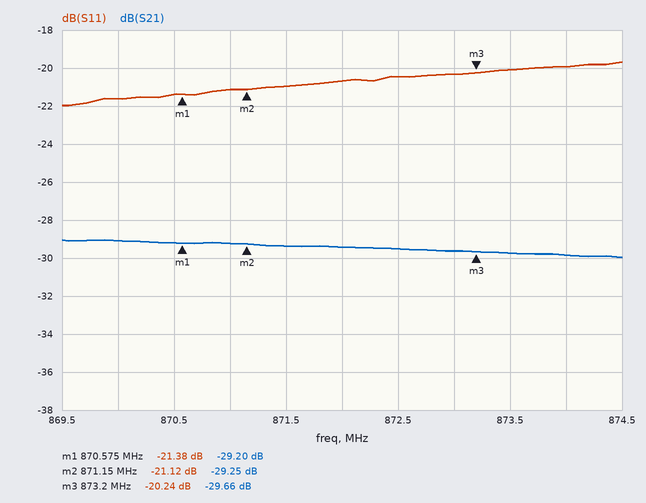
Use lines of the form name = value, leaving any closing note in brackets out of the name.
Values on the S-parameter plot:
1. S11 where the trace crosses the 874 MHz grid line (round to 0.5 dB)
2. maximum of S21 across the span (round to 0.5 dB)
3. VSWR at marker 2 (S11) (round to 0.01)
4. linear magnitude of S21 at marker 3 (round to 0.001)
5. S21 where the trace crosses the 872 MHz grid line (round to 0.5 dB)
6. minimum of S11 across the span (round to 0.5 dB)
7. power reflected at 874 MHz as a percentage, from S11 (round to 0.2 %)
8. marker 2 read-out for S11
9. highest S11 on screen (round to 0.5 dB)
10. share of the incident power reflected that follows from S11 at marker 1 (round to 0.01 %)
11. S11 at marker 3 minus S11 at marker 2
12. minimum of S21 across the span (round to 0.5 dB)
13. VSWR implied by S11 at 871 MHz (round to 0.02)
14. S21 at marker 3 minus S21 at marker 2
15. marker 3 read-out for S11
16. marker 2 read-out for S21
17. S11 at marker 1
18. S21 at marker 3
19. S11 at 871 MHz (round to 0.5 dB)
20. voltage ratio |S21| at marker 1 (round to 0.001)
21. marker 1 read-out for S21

S11 where the trace crosses the 874 MHz grid line = -20.0 dB
maximum of S21 across the span = -29.0 dB
VSWR at marker 2 (S11) = 1.19
linear magnitude of S21 at marker 3 = 0.033
S21 where the trace crosses the 872 MHz grid line = -29.5 dB
minimum of S11 across the span = -22.0 dB
power reflected at 874 MHz as a percentage, from S11 = 1.0 %
marker 2 read-out for S11 = -21.12 dB
highest S11 on screen = -19.5 dB
share of the incident power reflected that follows from S11 at marker 1 = 0.73 %
S11 at marker 3 minus S11 at marker 2 = 0.88 dB
minimum of S21 across the span = -30.0 dB
VSWR implied by S11 at 871 MHz = 1.20
S21 at marker 3 minus S21 at marker 2 = -0.41 dB
marker 3 read-out for S11 = -20.24 dB
marker 2 read-out for S21 = -29.25 dB
S11 at marker 1 = -21.38 dB
S21 at marker 3 = -29.66 dB
S11 at 871 MHz = -21.0 dB
voltage ratio |S21| at marker 1 = 0.035
marker 1 read-out for S21 = -29.20 dB
